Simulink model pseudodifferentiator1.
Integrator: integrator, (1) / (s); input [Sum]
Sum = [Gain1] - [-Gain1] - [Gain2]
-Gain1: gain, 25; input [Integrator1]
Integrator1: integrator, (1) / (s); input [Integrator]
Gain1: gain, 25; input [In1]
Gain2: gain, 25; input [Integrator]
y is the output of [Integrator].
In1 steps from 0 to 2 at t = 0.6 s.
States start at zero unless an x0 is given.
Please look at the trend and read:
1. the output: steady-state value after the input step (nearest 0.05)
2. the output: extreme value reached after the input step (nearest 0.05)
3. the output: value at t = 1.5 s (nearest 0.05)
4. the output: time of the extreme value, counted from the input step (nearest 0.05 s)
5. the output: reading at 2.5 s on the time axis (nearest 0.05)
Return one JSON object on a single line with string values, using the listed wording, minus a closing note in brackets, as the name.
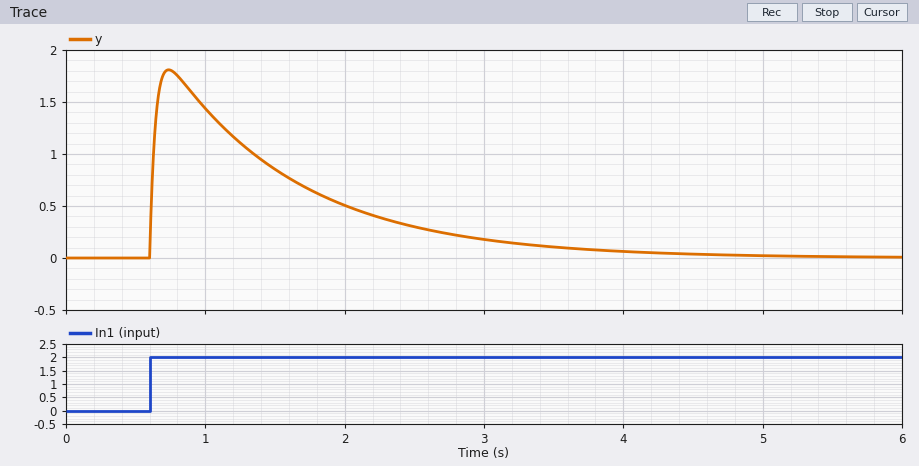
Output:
{"the output: steady-state value after the input step": "0.00", "the output: extreme value reached after the input step": "1.80", "the output: value at t = 1.5 s": "0.85", "the output: time of the extreme value, counted from the input step": "0.15 s", "the output: reading at 2.5 s on the time axis": "0.30"}
